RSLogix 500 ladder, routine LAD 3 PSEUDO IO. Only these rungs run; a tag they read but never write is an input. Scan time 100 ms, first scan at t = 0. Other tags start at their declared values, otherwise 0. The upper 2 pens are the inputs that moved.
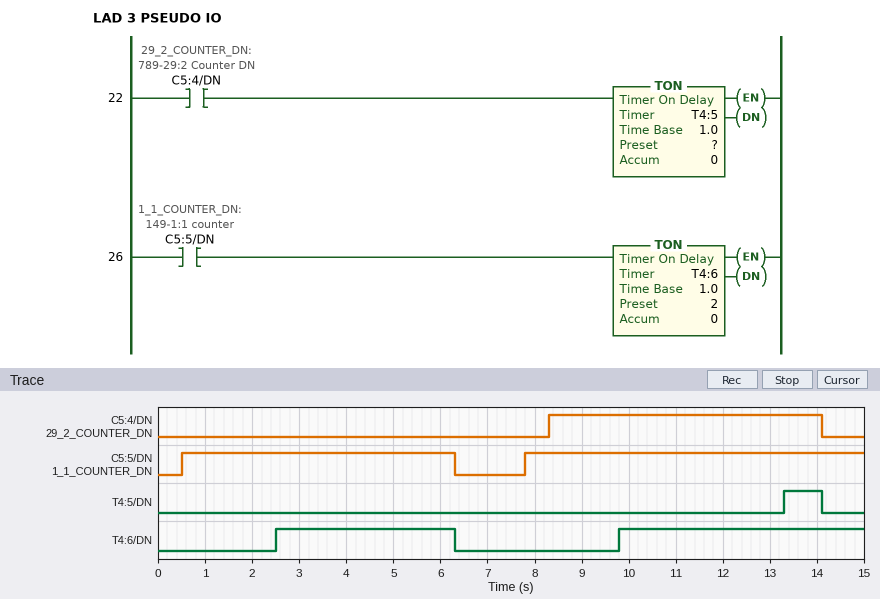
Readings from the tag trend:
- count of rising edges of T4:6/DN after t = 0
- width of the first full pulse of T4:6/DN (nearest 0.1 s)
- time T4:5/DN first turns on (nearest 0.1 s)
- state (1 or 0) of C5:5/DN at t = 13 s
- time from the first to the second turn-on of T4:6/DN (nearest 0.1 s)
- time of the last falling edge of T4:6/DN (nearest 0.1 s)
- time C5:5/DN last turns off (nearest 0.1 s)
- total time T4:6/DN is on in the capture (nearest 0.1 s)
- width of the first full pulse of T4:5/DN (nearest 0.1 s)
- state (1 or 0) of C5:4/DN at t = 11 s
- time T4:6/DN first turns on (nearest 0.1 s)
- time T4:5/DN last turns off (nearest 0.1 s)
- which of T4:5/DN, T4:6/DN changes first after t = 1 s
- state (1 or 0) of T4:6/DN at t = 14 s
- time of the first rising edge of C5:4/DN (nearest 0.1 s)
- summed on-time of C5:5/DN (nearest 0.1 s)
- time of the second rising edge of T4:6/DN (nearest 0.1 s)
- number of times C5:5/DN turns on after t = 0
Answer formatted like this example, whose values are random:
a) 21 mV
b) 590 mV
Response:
a) 2
b) 3.8 s
c) 13.3 s
d) 1
e) 7.3 s
f) 6.3 s
g) 6.3 s
h) 9.0 s
i) 0.8 s
j) 1
k) 2.5 s
l) 14.1 s
m) T4:6/DN
n) 1
o) 8.3 s
p) 13.0 s
q) 9.8 s
r) 2
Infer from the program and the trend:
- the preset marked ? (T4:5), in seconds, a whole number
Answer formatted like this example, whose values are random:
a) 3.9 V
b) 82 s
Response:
a) 5 s
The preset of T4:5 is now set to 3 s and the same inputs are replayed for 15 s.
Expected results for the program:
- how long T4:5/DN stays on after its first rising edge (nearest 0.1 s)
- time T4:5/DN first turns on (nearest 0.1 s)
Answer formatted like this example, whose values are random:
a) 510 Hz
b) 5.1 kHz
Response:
a) 2.8 s
b) 11.3 s
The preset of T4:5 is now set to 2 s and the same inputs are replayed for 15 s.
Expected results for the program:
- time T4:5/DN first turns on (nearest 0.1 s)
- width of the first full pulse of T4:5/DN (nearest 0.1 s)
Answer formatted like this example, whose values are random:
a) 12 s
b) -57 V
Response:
a) 10.3 s
b) 3.8 s
